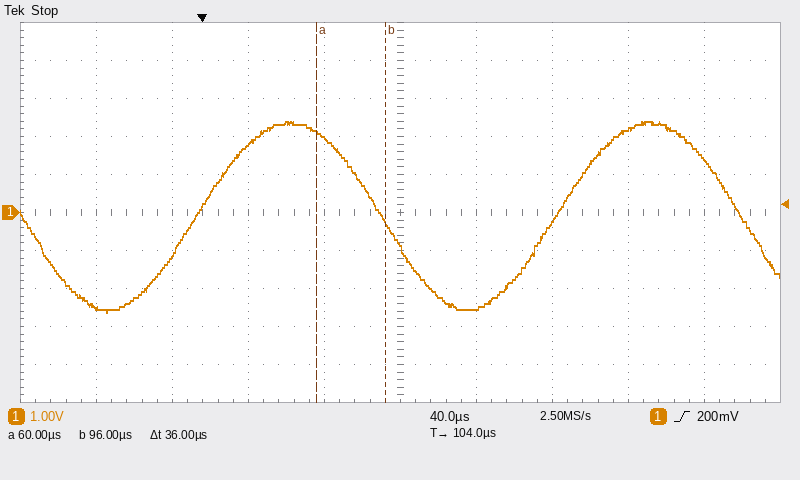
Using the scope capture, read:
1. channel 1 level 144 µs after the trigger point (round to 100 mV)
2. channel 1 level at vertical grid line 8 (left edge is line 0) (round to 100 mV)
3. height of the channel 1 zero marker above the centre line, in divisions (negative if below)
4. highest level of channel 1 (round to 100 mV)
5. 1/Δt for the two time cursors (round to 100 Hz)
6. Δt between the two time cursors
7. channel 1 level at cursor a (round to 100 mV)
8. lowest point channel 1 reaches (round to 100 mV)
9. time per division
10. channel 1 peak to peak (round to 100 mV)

-2.5 V
2.2 V
0.0 div
2.4 V
27.8 kHz
36 µs
2.1 V
-2.6 V
40 µs
5.0 V
